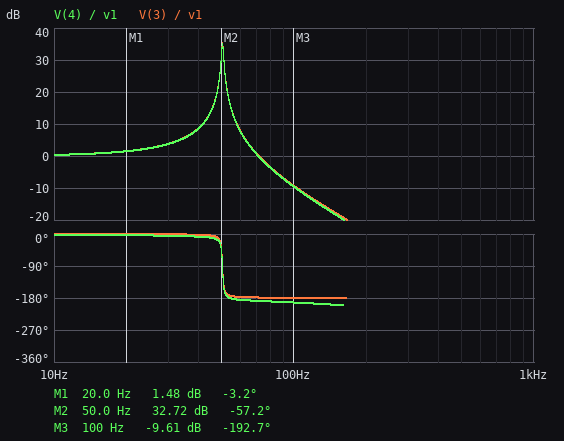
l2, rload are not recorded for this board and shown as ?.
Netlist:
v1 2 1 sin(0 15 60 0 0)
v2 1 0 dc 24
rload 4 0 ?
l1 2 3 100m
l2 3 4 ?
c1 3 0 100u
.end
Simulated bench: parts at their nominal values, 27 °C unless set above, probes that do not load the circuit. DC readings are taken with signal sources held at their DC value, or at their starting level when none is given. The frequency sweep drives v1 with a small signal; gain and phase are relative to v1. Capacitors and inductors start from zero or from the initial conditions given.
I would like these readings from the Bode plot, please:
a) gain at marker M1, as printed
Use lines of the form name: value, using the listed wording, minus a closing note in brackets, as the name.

gain at marker M1, as printed: 1.48 dB
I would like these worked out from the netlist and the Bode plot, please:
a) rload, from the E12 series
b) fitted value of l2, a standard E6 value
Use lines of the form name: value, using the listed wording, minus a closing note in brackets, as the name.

rload, from the E12 series: 1.8 kΩ
fitted value of l2, a standard E6 value: 680 mH
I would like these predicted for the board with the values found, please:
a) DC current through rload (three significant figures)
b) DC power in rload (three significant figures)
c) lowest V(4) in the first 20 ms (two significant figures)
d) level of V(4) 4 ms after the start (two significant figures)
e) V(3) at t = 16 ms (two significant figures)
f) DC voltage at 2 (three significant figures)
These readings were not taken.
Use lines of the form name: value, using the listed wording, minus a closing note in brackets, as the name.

DC current through rload: 13.3 mA
DC power in rload: 320 mW
lowest V(4) in the first 20 ms: -36 V
level of V(4) 4 ms after the start: 18 V
V(3) at t = 16 ms: -14 V
DC voltage at 2: 24.0 V
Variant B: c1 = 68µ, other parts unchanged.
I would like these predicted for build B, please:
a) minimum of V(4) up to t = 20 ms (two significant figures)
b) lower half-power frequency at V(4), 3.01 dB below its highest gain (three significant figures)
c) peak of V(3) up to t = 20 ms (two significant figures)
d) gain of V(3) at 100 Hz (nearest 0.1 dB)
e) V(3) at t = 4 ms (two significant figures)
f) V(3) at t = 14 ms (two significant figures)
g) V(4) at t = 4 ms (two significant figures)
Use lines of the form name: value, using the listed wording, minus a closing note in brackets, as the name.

minimum of V(4) up to t = 20 ms: -44 V
lower half-power frequency at V(4), 3.01 dB below its highest gain: 60.5 Hz
peak of V(3) up to t = 20 ms: 71 V
gain of V(3) at 100 Hz: -4.5 dB
V(3) at t = 4 ms: 30 V
V(3) at t = 14 ms: -18 V
V(4) at t = 4 ms: 25 V
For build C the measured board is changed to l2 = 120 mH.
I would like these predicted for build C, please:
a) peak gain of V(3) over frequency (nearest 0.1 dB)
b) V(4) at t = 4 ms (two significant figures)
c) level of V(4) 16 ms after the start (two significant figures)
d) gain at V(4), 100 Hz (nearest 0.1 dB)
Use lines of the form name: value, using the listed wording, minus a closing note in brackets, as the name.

peak gain of V(3) over frequency: 35.1 dB
V(4) at t = 4 ms: 21 V
level of V(4) 16 ms after the start: -13 V
gain at V(4), 100 Hz: -9.4 dB
